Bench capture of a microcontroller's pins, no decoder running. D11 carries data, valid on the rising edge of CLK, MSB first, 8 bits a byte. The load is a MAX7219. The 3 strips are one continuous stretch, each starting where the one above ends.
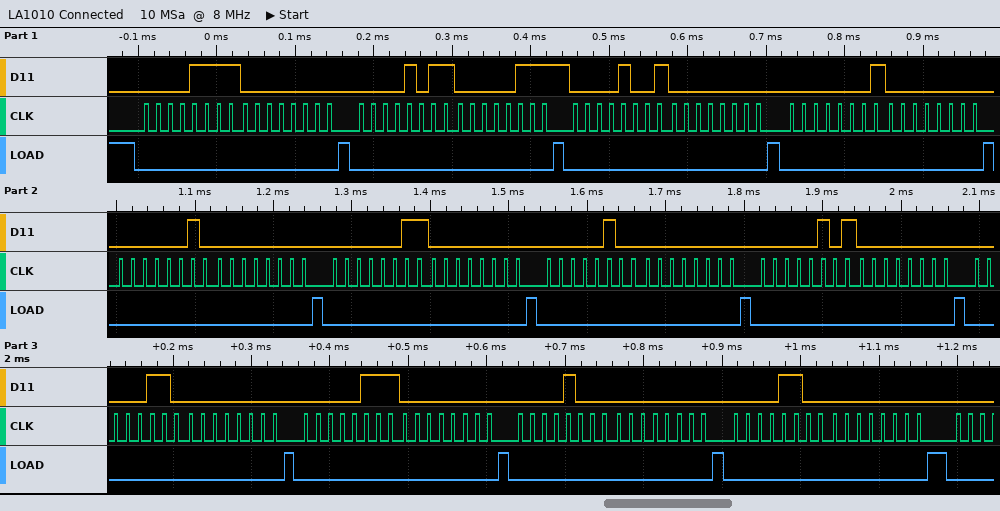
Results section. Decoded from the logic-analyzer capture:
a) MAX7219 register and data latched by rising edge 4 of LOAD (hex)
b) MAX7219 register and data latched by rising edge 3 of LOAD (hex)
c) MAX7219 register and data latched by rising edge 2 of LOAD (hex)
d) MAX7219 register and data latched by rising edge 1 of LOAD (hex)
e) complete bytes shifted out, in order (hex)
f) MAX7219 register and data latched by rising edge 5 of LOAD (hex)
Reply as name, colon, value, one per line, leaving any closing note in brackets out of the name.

MAX7219 register and data latched by rising edge 4 of LOAD: register 0x1, data 0x00
MAX7219 register and data latched by rising edge 3 of LOAD: register 0x9, data 0x00
MAX7219 register and data latched by rising edge 2 of LOAD: register 0xB, data 0x07
MAX7219 register and data latched by rising edge 1 of LOAD: register 0xF, data 0x00
complete bytes shifted out, in order: 0F 00 0B 07 09 00 01 00 02 00 03 00 04 00 05 00 06 00 07 00 08 00 0C 00
MAX7219 register and data latched by rising edge 5 of LOAD: register 0x2, data 0x00
